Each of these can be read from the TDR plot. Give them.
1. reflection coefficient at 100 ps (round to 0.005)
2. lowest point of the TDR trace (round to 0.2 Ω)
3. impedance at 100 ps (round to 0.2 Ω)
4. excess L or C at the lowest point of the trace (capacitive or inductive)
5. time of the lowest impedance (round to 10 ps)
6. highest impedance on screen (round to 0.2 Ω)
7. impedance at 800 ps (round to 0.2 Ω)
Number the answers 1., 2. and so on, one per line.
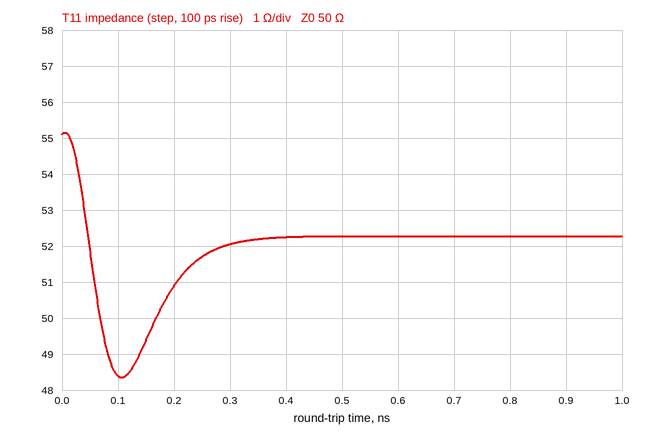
1. -0.015
2. 48.4 Ω
3. 48.4 Ω
4. capacitive
5. 110 ps
6. 55.2 Ω
7. 52.2 Ω
